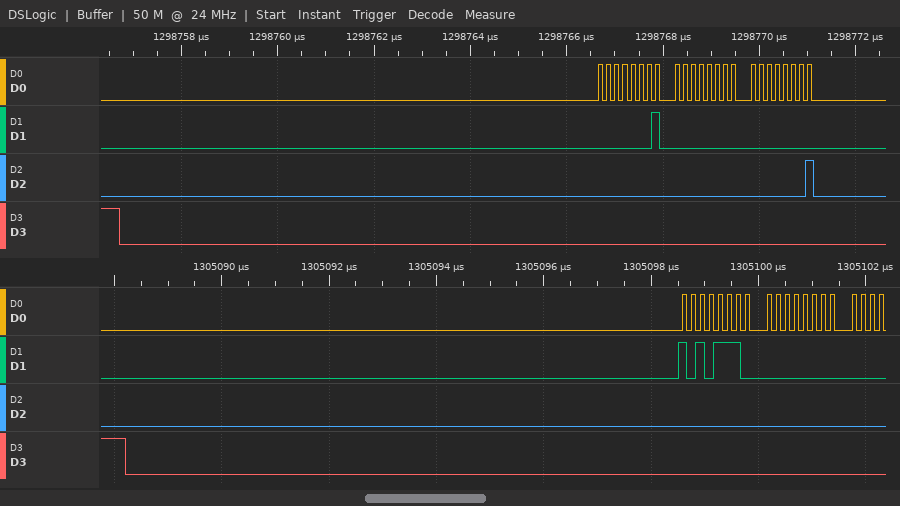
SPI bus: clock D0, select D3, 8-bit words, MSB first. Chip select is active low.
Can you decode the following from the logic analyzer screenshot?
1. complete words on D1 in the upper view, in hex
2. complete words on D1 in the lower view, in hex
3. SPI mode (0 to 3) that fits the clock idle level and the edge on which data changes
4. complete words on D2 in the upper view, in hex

01, 00, 00
AE, 00
0
00, 00, 01
